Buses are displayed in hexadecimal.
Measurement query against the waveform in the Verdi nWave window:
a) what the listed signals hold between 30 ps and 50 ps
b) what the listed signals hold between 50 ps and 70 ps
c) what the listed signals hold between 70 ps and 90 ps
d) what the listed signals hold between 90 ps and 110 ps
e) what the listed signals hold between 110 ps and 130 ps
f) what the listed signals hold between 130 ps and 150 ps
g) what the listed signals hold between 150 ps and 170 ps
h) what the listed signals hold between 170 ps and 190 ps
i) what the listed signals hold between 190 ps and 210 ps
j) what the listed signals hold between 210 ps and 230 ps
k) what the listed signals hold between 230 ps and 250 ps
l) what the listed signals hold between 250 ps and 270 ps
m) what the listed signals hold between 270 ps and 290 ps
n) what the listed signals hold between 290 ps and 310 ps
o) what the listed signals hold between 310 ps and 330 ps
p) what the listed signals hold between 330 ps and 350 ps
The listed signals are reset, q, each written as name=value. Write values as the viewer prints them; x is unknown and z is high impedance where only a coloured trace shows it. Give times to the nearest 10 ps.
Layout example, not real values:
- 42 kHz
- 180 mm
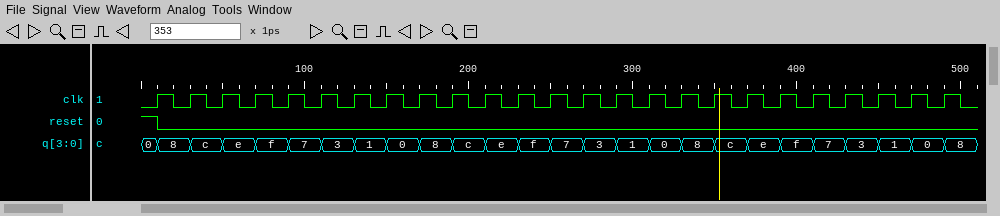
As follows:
- reset=0, q=c
- reset=0, q=e
- reset=0, q=f
- reset=0, q=7
- reset=0, q=3
- reset=0, q=1
- reset=0, q=0
- reset=0, q=8
- reset=0, q=c
- reset=0, q=e
- reset=0, q=f
- reset=0, q=7
- reset=0, q=3
- reset=0, q=1
- reset=0, q=0
- reset=0, q=8
